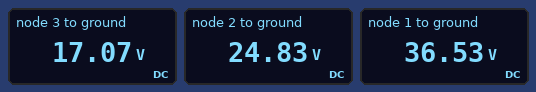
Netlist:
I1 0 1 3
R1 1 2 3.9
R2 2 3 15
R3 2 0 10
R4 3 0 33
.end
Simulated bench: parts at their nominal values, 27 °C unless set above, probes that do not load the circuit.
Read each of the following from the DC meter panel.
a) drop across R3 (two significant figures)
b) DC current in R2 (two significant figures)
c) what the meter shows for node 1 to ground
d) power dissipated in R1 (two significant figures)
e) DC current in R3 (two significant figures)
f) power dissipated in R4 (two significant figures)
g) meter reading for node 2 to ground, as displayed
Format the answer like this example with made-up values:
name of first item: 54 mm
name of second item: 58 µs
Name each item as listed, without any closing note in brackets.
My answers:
drop across R3: 25 V
DC current in R2: 520 mA
what the meter shows for node 1 to ground: 36.53 V
power dissipated in R1: 35 W
DC current in R3: 2.5 A
power dissipated in R4: 8.8 W
meter reading for node 2 to ground, as displayed: 24.83 V
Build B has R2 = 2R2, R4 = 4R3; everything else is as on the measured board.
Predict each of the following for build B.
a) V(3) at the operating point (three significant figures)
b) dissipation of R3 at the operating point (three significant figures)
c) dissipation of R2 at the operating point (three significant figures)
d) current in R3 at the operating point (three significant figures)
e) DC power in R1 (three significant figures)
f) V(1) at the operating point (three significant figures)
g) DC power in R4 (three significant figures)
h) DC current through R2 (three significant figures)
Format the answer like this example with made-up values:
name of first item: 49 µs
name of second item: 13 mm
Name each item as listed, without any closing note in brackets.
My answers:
V(3) at the operating point: 7.82 V
dissipation of R3 at the operating point: 14.0 W
dissipation of R2 at the operating point: 7.27 W
current in R3 at the operating point: 1.18 A
DC power in R1: 35.1 W
V(1) at the operating point: 23.5 V
DC power in R4: 14.2 W
DC current through R2: 1.82 A
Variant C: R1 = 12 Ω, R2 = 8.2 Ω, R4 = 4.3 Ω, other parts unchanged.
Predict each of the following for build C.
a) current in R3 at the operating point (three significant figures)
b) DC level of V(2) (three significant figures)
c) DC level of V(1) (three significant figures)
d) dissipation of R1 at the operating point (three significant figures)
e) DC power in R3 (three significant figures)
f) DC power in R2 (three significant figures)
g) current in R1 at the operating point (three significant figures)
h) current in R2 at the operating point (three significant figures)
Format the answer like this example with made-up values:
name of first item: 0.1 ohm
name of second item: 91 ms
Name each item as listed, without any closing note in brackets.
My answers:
current in R3 at the operating point: 1.67 A
DC level of V(2): 16.7 V
DC level of V(1): 52.7 V
dissipation of R1 at the operating point: 108 W
DC power in R3: 27.8 W
DC power in R2: 14.6 W
current in R1 at the operating point: 3.00 A
current in R2 at the operating point: 1.33 A
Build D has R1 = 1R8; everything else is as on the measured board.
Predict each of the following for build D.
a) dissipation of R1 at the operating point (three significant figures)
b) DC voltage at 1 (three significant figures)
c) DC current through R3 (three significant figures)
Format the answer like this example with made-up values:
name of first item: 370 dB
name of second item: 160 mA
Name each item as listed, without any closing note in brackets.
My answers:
dissipation of R1 at the operating point: 16.2 W
DC voltage at 1: 30.2 V
DC current through R3: 2.48 A
